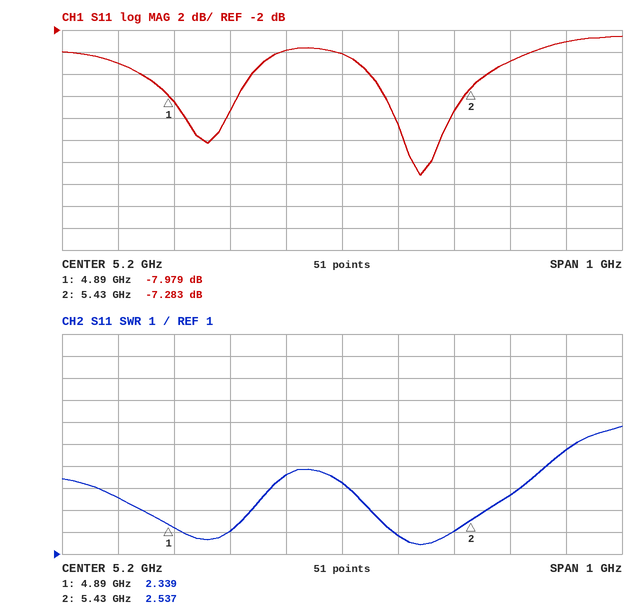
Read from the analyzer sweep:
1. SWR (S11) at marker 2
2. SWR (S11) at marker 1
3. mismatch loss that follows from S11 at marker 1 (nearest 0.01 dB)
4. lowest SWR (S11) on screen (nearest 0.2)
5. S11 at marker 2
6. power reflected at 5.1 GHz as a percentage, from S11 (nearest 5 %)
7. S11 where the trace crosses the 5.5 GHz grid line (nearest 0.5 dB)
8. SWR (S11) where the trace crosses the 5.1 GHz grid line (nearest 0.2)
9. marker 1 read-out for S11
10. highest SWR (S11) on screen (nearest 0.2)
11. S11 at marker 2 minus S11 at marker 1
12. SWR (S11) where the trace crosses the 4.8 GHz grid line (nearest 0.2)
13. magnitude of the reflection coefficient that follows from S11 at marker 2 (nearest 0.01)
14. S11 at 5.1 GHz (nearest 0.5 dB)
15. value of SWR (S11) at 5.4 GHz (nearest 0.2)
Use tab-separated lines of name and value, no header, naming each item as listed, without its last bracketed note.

SWR (S11) at marker 2	2.537
SWR (S11) at marker 1	2.339
mismatch loss that follows from S11 at marker 1	0.75 dB
lowest SWR (S11) on screen	1.4
S11 at marker 2	-7.283 dB
power reflected at 5.1 GHz as a percentage, from S11	40 %
S11 where the trace crosses the 5.5 GHz grid line	-5.0 dB
SWR (S11) where the trace crosses the 5.1 GHz grid line	4.6
marker 1 read-out for S11	-7.979 dB
highest SWR (S11) on screen	6.8
S11 at marker 2 minus S11 at marker 1	0.696 dB
SWR (S11) where the trace crosses the 4.8 GHz grid line	3.6
magnitude of the reflection coefficient that follows from S11 at marker 2	0.43
S11 at 5.1 GHz	-4.0 dB
value of SWR (S11) at 5.4 GHz	2.0
